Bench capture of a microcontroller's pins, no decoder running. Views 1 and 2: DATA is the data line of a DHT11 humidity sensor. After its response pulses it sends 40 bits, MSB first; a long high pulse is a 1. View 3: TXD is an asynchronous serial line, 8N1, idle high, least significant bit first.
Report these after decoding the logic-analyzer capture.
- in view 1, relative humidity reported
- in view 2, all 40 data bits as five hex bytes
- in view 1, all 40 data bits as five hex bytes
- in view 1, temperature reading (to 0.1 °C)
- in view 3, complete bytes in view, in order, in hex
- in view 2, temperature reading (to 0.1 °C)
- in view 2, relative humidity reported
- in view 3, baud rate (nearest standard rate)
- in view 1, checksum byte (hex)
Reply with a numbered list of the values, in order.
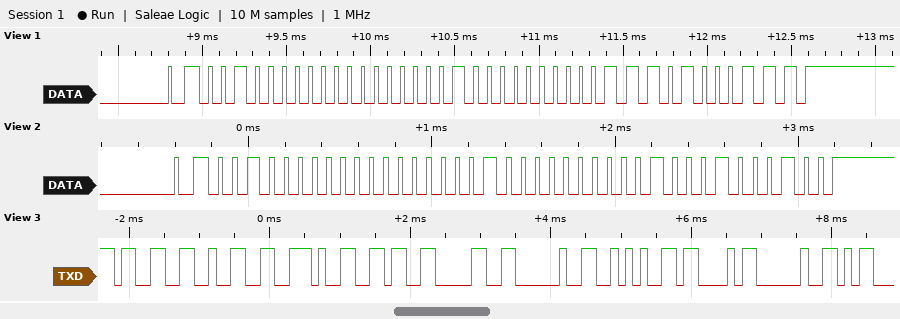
1. 32 %
2. 20 00 20 04 44
3. 20 00 20 07 47
4. 32.7 °C
5. 33 32 2E 36 30 20 2A 43 20
6. 32.4 °C
7. 32 %
8. 9600 baud
9. 0x47
